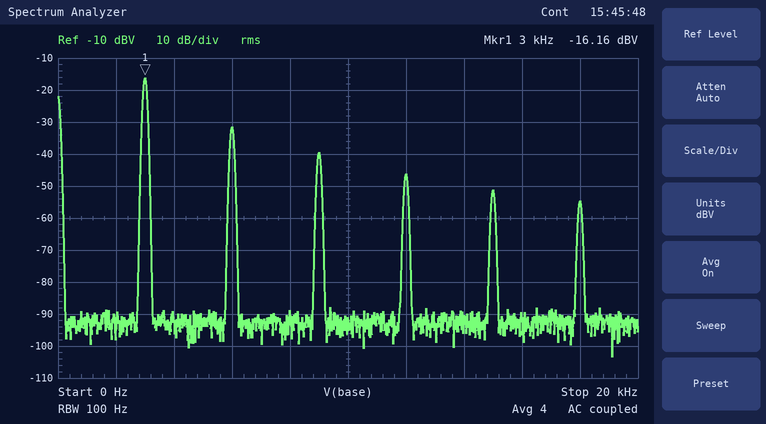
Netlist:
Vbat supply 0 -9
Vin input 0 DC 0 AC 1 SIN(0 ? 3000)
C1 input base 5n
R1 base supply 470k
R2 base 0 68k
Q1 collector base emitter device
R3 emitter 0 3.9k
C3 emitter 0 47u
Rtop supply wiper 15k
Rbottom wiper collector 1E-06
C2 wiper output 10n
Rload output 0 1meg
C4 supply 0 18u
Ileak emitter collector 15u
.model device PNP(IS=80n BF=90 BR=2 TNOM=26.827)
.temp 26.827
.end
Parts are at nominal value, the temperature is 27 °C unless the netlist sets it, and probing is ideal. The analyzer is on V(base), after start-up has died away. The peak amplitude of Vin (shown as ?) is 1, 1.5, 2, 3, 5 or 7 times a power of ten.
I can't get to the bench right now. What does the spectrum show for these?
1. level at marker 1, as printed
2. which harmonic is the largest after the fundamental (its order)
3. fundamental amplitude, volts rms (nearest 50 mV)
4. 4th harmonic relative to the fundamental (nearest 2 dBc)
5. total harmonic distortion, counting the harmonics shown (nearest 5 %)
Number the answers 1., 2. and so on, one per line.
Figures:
1. -16.16 dBV
2. 2
3. 150 mV
4. -30 dBc
5. 20 %
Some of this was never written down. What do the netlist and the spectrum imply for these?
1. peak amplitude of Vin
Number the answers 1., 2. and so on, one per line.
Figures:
1. 300 mV
